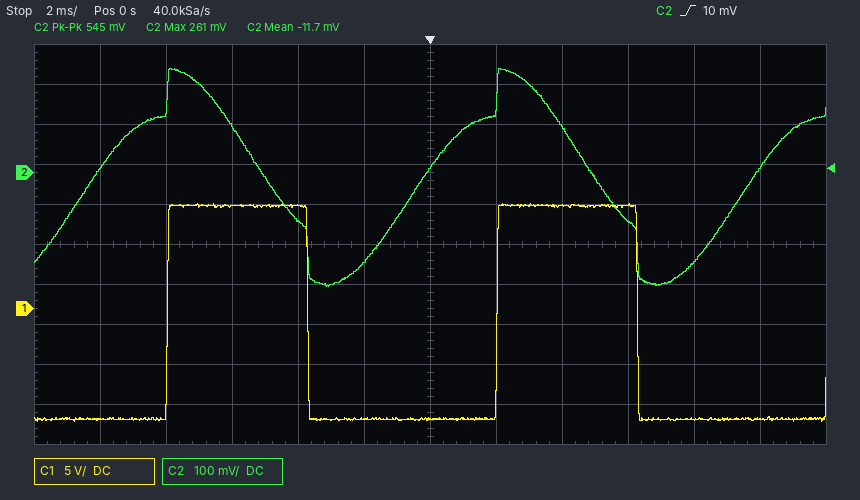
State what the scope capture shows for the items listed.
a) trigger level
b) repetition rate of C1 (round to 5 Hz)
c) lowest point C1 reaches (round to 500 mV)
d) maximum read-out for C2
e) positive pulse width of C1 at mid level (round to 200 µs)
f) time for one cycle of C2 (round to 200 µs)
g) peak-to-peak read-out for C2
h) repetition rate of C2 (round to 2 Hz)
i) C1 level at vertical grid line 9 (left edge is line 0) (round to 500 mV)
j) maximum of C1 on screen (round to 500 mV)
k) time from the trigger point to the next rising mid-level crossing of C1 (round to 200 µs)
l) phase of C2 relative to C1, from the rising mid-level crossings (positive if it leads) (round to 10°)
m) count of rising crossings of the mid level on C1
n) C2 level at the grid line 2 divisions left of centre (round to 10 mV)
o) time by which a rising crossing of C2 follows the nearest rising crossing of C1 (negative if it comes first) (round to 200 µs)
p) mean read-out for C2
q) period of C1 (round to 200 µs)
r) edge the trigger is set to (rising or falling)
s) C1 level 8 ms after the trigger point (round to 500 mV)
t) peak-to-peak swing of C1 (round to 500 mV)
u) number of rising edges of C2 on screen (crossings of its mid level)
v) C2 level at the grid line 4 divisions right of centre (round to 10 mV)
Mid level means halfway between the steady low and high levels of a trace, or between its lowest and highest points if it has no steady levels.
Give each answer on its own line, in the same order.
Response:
10 mV
100 Hz
-14.0 V
261 mV
4.2 ms
10.0 ms
545 mV
100 Hz
13.0 V
13.0 V
2.0 ms
+80°
2
-120 mV
-2.2 ms
-11.7 mV
10.0 ms
rising
-14.0 V
27.0 V
3
-220 mV
